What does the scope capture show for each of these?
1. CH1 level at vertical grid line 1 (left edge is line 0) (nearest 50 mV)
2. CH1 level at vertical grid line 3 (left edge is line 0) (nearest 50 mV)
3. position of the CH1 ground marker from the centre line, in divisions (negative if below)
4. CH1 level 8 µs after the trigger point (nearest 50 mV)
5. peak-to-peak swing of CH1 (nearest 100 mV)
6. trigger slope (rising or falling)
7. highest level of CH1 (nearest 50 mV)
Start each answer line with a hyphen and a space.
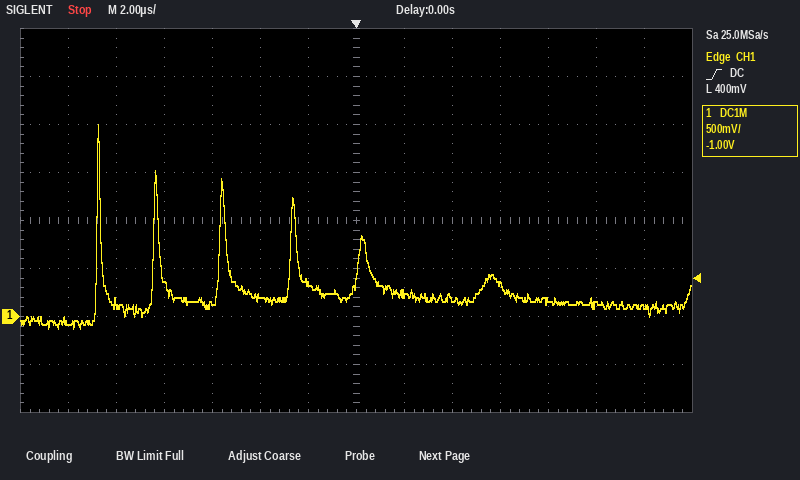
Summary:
- -50 mV
- 400 mV
- -2.0 div
- 150 mV
- 2.10 V
- rising
- 2.00 V
